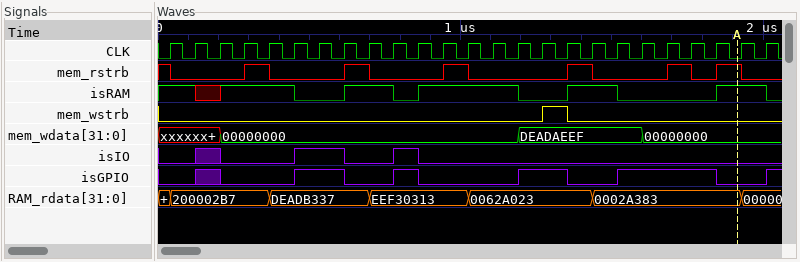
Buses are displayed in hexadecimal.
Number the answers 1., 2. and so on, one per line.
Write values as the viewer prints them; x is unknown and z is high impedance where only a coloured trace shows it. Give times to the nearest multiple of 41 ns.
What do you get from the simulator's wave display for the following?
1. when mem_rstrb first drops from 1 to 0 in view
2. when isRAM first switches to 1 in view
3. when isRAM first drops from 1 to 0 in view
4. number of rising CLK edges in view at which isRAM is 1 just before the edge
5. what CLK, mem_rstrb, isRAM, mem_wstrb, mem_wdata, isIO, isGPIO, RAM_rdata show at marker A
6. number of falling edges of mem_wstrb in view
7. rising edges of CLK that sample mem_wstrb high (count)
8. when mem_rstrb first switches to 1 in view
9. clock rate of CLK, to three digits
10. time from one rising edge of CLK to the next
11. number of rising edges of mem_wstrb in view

1. 41 ns
2. 205 ns
3. 451 ns
4. 15
5. CLK=0, mem_rstrb=1, isRAM=1, mem_wstrb=0, mem_wdata=00000000, isIO=0, isGPIO=0, RAM_rdata=0002A383
6. 1
7. 1
8. 287 ns
9. 12.2 MHz
10. 82 ns
11. 1
